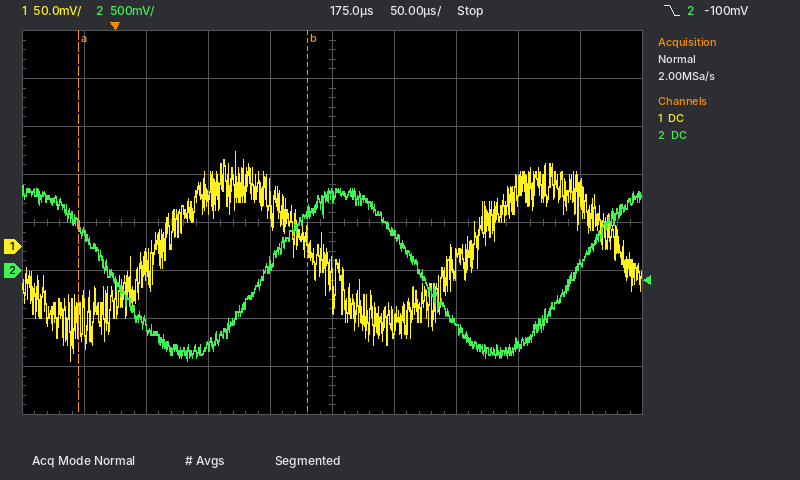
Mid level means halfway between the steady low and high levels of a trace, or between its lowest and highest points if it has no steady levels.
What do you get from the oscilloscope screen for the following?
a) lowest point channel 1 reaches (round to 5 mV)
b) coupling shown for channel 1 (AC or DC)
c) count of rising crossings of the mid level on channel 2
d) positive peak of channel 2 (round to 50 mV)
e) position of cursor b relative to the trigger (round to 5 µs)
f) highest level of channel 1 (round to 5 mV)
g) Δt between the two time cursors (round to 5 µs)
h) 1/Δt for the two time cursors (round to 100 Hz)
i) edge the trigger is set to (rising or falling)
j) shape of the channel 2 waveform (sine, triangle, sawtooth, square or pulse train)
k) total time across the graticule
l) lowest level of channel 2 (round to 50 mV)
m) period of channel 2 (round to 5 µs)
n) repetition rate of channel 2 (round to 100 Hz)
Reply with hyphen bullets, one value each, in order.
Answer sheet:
- -120 mV
- DC
- 2
- 900 mV
- +155 µs
- 100 mV
- 185 µs
- 5.4 kHz
- falling
- sine
- 500 µs
- -950 mV
- 250 µs
- 4.0 kHz
